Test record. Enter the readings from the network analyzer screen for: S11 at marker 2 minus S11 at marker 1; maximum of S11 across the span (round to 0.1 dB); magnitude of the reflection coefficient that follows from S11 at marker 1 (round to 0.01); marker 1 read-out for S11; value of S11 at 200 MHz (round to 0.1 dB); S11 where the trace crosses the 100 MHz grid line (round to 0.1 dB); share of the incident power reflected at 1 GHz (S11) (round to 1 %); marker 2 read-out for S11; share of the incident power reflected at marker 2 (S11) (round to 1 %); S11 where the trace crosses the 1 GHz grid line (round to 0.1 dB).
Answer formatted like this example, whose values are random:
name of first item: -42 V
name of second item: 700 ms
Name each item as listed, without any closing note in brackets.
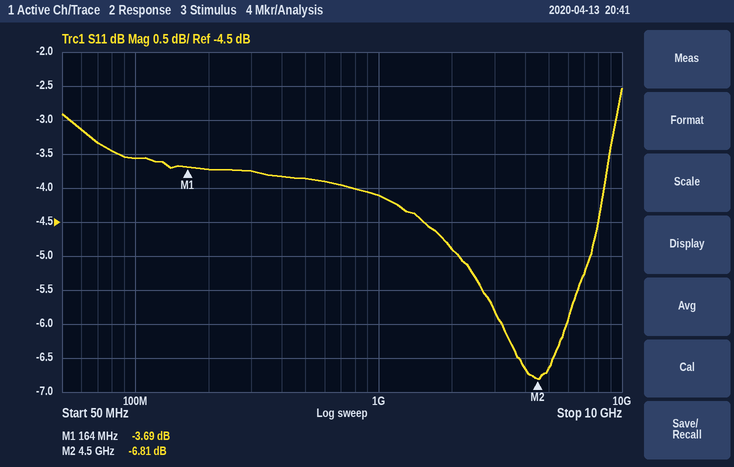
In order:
S11 at marker 2 minus S11 at marker 1: -3.12 dB
maximum of S11 across the span: -2.5 dB
magnitude of the reflection coefficient that follows from S11 at marker 1: 0.65
marker 1 read-out for S11: -3.69 dB
value of S11 at 200 MHz: -3.7 dB
S11 where the trace crosses the 100 MHz grid line: -3.6 dB
share of the incident power reflected at 1 GHz (S11): 39 %
marker 2 read-out for S11: -6.81 dB
share of the incident power reflected at marker 2 (S11): 21 %
S11 where the trace crosses the 1 GHz grid line: -4.1 dB
